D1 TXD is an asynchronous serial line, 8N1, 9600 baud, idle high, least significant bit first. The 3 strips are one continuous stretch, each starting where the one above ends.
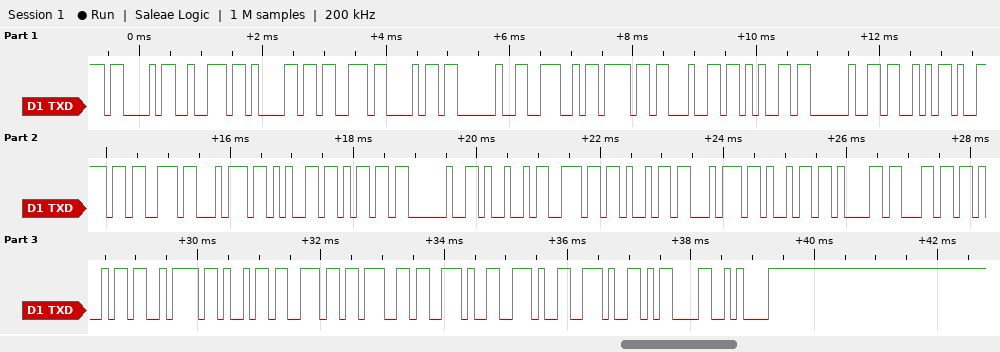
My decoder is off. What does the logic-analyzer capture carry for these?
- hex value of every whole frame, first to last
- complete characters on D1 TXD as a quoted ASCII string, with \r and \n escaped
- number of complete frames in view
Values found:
43 72 61 73 68 20 4E 6F 64 65 20 53 79 73 74 65 6D 20 49 6E 69 74 69 61 6C 69 7A 69 6E 67 2E 2E 2E 0D 0A
"Crash Node System Initializing...\r\n"
35
